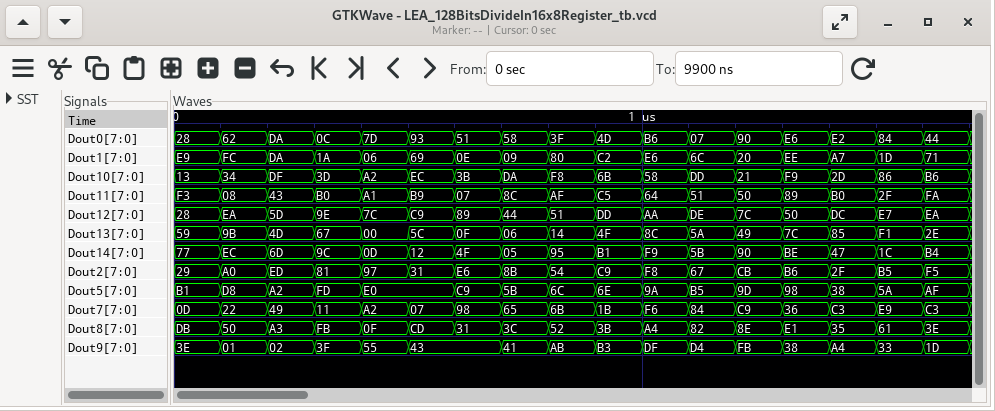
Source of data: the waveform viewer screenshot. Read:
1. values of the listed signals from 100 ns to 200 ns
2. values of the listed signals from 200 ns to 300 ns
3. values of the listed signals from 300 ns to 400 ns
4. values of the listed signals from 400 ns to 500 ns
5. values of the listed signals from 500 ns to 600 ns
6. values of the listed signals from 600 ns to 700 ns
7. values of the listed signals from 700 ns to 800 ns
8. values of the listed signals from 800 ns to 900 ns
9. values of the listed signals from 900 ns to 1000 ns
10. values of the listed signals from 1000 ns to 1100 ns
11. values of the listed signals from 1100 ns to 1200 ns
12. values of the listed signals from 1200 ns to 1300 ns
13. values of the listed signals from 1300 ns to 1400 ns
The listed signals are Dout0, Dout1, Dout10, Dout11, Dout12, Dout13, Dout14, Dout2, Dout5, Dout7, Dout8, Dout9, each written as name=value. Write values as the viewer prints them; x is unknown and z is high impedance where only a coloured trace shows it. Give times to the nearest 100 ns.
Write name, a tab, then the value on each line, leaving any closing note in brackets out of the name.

values of the listed signals from 100 ns to 200 ns	Dout0=62, Dout1=FC, Dout10=34, Dout11=08, Dout12=EA, Dout13=9B, Dout14=EC, Dout2=A0, Dout5=D8, Dout7=22, Dout8=50, Dout9=01
values of the listed signals from 200 ns to 300 ns	Dout0=DA, Dout1=DA, Dout10=DF, Dout11=43, Dout12=5D, Dout13=4D, Dout14=6D, Dout2=ED, Dout5=A2, Dout7=49, Dout8=A3, Dout9=02
values of the listed signals from 300 ns to 400 ns	Dout0=0C, Dout1=1A, Dout10=3D, Dout11=B0, Dout12=9E, Dout13=67, Dout14=9C, Dout2=81, Dout5=FD, Dout7=11, Dout8=FB, Dout9=3F
values of the listed signals from 400 ns to 500 ns	Dout0=7D, Dout1=06, Dout10=A2, Dout11=A1, Dout12=7C, Dout13=00, Dout14=0D, Dout2=97, Dout5=E0, Dout7=A2, Dout8=0F, Dout9=55
values of the listed signals from 500 ns to 600 ns	Dout0=93, Dout1=69, Dout10=EC, Dout11=B9, Dout12=C9, Dout13=5C, Dout14=12, Dout2=31, Dout5=E0, Dout7=07, Dout8=CD, Dout9=43
values of the listed signals from 600 ns to 700 ns	Dout0=51, Dout1=0E, Dout10=3B, Dout11=07, Dout12=89, Dout13=0F, Dout14=4F, Dout2=E6, Dout5=C9, Dout7=98, Dout8=31, Dout9=43
values of the listed signals from 700 ns to 800 ns	Dout0=58, Dout1=09, Dout10=DA, Dout11=8C, Dout12=44, Dout13=06, Dout14=05, Dout2=8B, Dout5=5B, Dout7=65, Dout8=3C, Dout9=41
values of the listed signals from 800 ns to 900 ns	Dout0=3F, Dout1=80, Dout10=F8, Dout11=AF, Dout12=51, Dout13=14, Dout14=95, Dout2=54, Dout5=6C, Dout7=6B, Dout8=52, Dout9=AB
values of the listed signals from 900 ns to 1000 ns	Dout0=4D, Dout1=C2, Dout10=6B, Dout11=C5, Dout12=DD, Dout13=4F, Dout14=B1, Dout2=C9, Dout5=6E, Dout7=1B, Dout8=3B, Dout9=B3
values of the listed signals from 1000 ns to 1100 ns	Dout0=B6, Dout1=E6, Dout10=58, Dout11=64, Dout12=AA, Dout13=8C, Dout14=F9, Dout2=F8, Dout5=9A, Dout7=F6, Dout8=A4, Dout9=DF
values of the listed signals from 1100 ns to 1200 ns	Dout0=07, Dout1=6C, Dout10=DD, Dout11=51, Dout12=DE, Dout13=5A, Dout14=5B, Dout2=67, Dout5=B5, Dout7=84, Dout8=82, Dout9=D4
values of the listed signals from 1200 ns to 1300 ns	Dout0=90, Dout1=20, Dout10=21, Dout11=50, Dout12=7C, Dout13=49, Dout14=90, Dout2=CB, Dout5=9D, Dout7=C9, Dout8=8E, Dout9=FB
values of the listed signals from 1300 ns to 1400 ns	Dout0=E6, Dout1=EE, Dout10=F9, Dout11=89, Dout12=50, Dout13=7C, Dout14=BE, Dout2=B6, Dout5=98, Dout7=36, Dout8=E1, Dout9=38
